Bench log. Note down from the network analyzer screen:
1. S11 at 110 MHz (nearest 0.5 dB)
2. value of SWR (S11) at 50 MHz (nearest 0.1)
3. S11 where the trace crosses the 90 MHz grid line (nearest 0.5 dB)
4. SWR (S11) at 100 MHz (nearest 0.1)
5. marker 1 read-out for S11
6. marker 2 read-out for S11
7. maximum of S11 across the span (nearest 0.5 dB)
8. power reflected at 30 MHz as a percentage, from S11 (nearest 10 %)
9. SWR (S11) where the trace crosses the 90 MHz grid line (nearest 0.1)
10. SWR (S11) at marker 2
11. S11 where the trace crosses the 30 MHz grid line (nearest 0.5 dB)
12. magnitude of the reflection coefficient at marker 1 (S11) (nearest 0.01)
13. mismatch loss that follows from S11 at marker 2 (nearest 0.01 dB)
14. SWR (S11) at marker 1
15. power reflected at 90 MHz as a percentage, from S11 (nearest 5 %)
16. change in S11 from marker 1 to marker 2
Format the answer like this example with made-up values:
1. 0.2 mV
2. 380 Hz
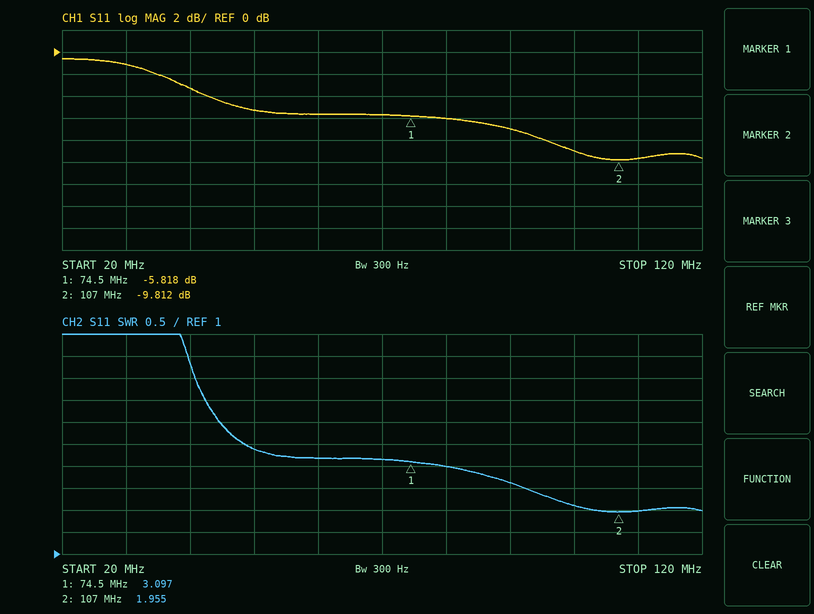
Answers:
1. -9.5 dB
2. 3.4
3. -7.0 dB
4. 2.1
5. -5.818 dB
6. -9.812 dB
7. -0.5 dB
8. 80 %
9. 2.6
10. 1.955
11. -1.0 dB
12. 0.51
13. 0.48 dB
14. 3.097
15. 20 %
16. -3.994 dB
